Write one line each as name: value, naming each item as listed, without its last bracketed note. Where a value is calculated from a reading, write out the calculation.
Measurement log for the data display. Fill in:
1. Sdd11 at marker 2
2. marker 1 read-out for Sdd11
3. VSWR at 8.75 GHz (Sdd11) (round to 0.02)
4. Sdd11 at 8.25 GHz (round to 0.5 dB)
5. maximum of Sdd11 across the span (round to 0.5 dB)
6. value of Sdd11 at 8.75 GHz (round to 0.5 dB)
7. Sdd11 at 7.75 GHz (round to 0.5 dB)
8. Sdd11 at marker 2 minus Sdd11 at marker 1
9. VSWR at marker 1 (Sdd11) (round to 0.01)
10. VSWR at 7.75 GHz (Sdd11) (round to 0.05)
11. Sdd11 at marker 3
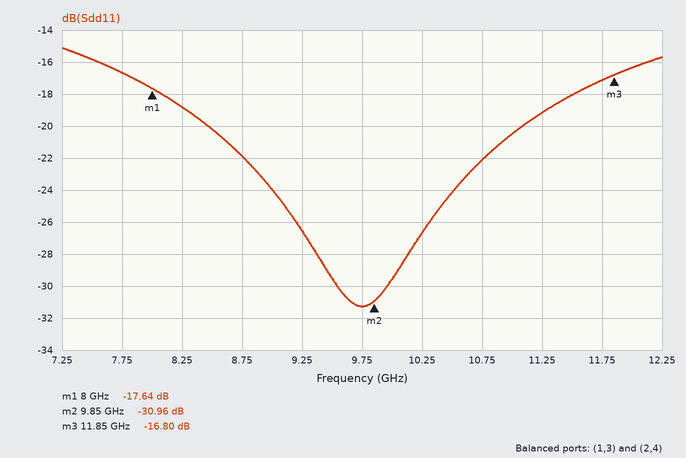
Sdd11 at marker 2: -30.96 dB
marker 1 read-out for Sdd11: -17.64 dB
VSWR at 8.75 GHz (Sdd11): |Γ| = 10^(-22/20) = 0.0794; VSWR = (1 + 0.0794)/(1 − 0.0794) ≈ 1.17, so 1.18 to the nearest 0.02
Sdd11 at 8.25 GHz: -19.0 dB
maximum of Sdd11 across the span: -15.0 dB
value of Sdd11 at 8.75 GHz: -22.0 dB
Sdd11 at 7.75 GHz: -16.5 dB
Sdd11 at marker 2 minus Sdd11 at marker 1: -30.96 − (-17.64) = -13.32 dB
VSWR at marker 1 (Sdd11): (1 + 0.1312)/(1 − 0.1312) ≈ 1.30
VSWR at 7.75 GHz (Sdd11): |Γ| = 10^(-16.5/20) = 0.1496; VSWR = (1 + 0.1496)/(1 − 0.1496) ≈ 1.35
Sdd11 at marker 3: -16.80 dB
